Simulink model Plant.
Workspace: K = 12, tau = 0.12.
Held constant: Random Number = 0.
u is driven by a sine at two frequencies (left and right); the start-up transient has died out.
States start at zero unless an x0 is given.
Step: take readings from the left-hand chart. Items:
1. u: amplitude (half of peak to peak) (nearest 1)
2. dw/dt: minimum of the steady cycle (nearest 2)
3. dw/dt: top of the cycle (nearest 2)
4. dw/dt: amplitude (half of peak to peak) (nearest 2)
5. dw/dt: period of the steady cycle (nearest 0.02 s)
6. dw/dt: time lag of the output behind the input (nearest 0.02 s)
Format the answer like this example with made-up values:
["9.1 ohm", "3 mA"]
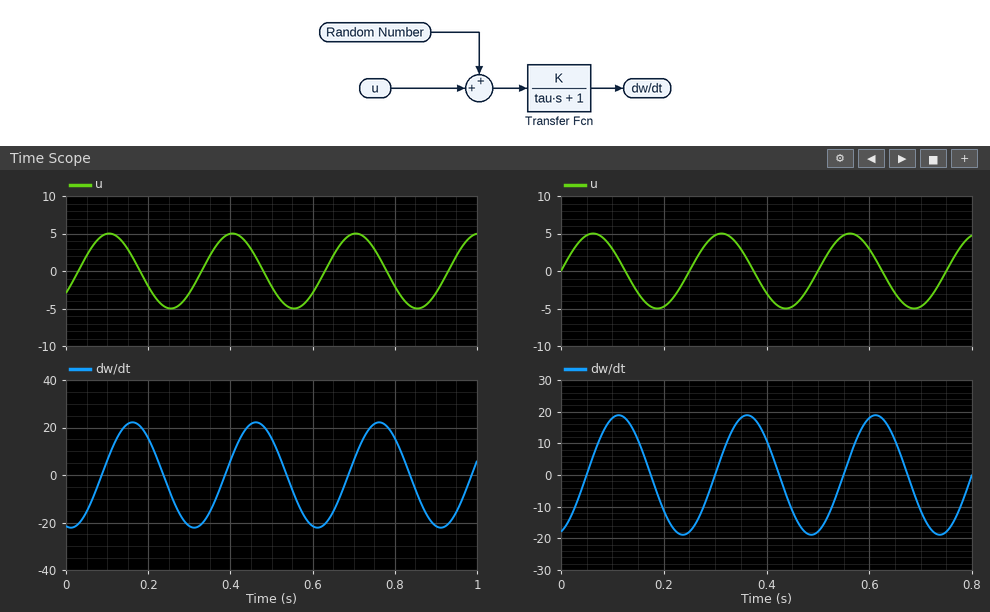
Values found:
["5", "-22", "22", "22", "0.30 s", "0.06 s"]
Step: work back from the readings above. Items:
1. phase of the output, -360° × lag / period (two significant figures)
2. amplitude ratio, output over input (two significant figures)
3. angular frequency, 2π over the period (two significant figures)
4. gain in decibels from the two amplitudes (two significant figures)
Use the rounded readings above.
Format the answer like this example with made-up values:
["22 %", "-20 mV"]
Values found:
["-72°", "4.4", "21 rad/s", "13 dB"]
